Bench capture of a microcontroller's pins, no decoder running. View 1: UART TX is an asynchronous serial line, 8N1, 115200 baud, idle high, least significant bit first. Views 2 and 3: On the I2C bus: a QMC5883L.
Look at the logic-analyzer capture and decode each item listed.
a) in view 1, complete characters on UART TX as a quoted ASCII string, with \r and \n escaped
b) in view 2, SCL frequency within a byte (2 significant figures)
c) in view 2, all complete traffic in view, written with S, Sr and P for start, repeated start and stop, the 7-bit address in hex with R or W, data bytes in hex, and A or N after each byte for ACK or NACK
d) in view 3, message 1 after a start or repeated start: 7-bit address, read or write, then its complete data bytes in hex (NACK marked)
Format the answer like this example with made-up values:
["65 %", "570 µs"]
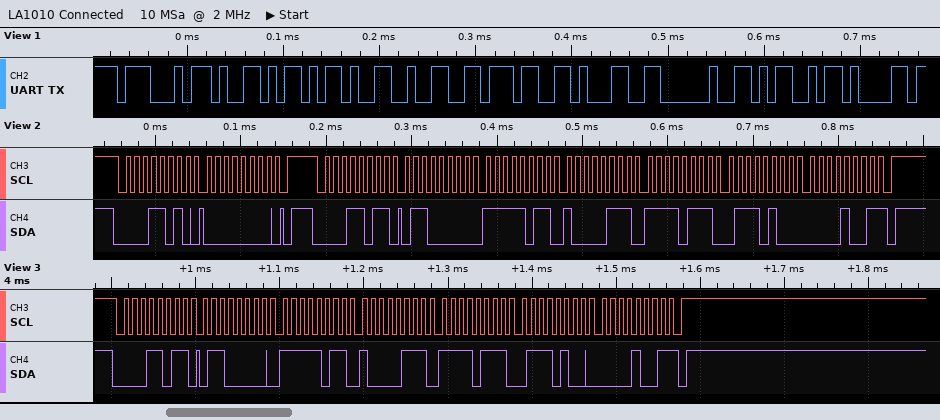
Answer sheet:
["\"GY-271 Ma\"", "100 kHz", "S 0DW A 00 A P S 0DR A 60 A FB A 87 A F7 A 74 A 09 N P", "0x0D read: 60 FB 87 F7 74 09 NACK"]
